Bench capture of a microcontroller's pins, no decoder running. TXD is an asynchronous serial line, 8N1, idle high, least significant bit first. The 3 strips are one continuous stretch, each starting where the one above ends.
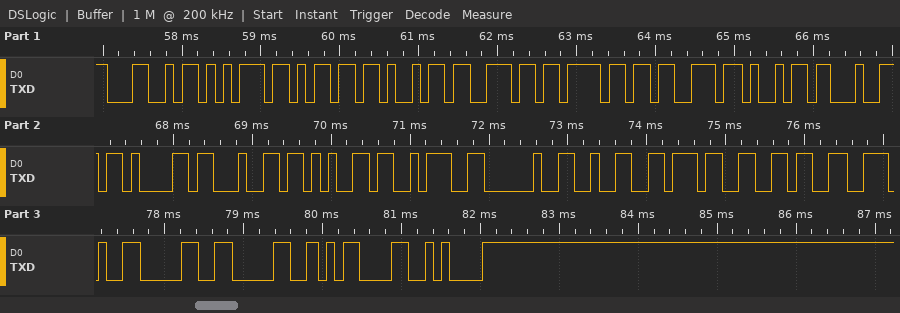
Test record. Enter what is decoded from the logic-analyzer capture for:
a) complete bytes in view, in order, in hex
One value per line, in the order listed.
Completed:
4C 75 6D 69 6E 6F 73 69 64 61 64 65 3A 20 32 37 36 2E 30 30 0D 0A
